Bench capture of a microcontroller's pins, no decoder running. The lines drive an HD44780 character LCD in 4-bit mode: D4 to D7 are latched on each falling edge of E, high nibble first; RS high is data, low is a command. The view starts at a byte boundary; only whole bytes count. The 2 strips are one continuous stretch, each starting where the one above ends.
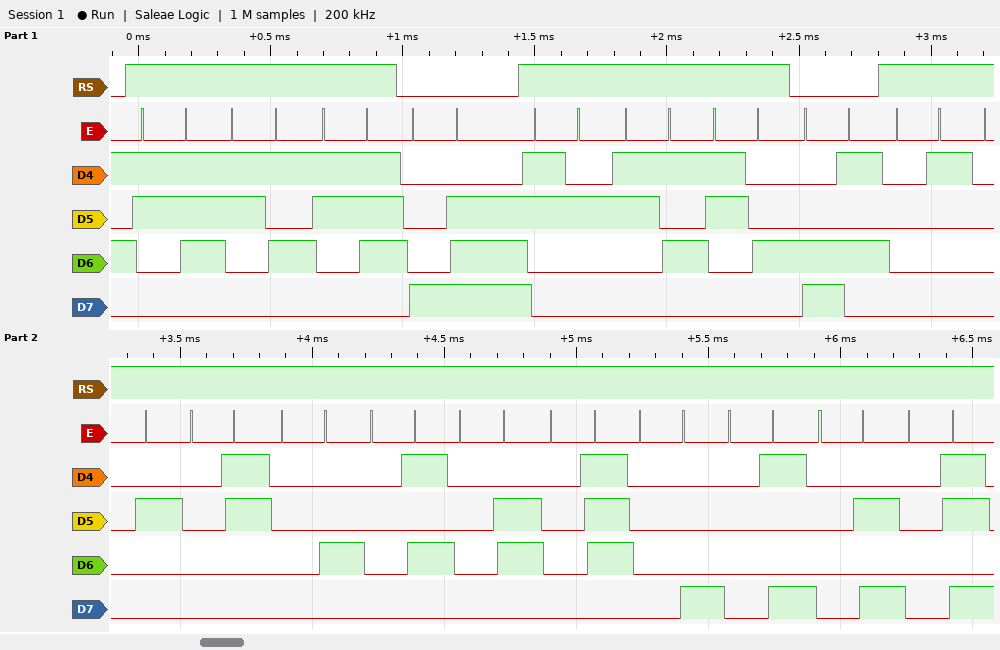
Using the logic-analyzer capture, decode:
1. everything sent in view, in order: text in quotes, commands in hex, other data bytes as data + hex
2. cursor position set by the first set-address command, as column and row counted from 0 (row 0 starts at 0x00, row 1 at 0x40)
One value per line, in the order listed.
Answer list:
"757" 0x8E "254" 0xC5 data 01 02 03 04 05 06 07 08 09 0A 0B
column 14, row 0
